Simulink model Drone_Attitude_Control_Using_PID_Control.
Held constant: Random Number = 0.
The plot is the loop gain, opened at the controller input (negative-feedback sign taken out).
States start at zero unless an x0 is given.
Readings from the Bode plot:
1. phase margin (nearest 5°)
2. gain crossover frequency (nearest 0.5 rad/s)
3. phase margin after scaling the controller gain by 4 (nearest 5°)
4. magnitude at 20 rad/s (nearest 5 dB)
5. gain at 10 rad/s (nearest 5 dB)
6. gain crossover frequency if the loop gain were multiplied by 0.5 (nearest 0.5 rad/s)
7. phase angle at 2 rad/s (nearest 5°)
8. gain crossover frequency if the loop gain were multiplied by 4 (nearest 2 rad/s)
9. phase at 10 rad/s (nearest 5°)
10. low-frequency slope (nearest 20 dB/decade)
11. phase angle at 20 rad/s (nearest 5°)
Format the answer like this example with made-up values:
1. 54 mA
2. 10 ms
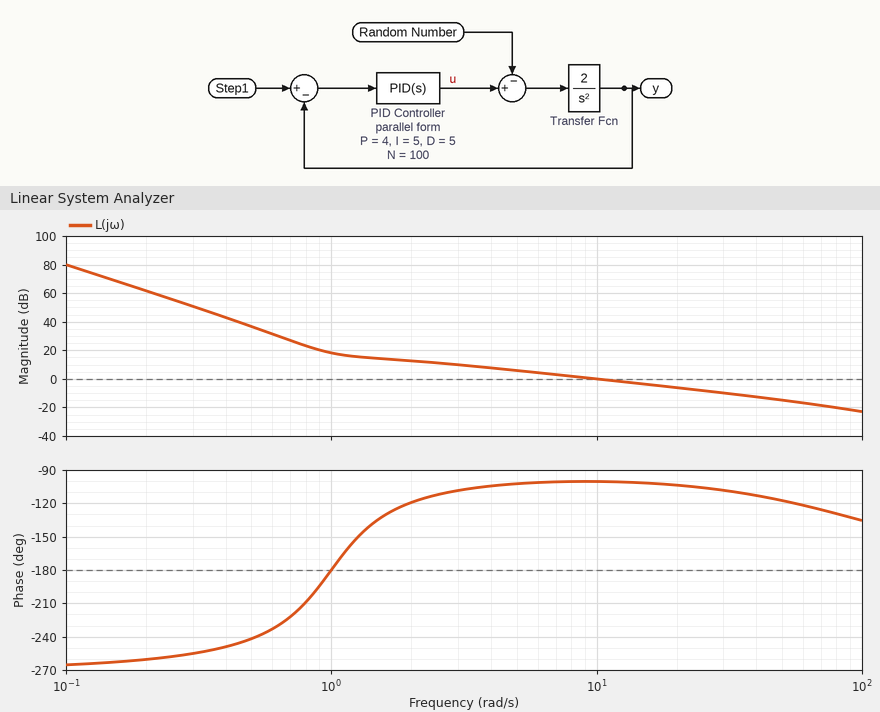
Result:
1. 80°
2. 10.0 rad/s
3. 70°
4. -5 dB
5. 0 dB
6. 5.0 rad/s
7. -120°
8. 38 rad/s
9. -100°
10. -60 dB/decade
11. -105°
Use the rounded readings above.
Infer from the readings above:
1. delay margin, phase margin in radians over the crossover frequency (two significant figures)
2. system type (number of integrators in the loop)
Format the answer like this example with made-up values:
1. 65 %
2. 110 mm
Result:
1. 0.14 s
2. 3
